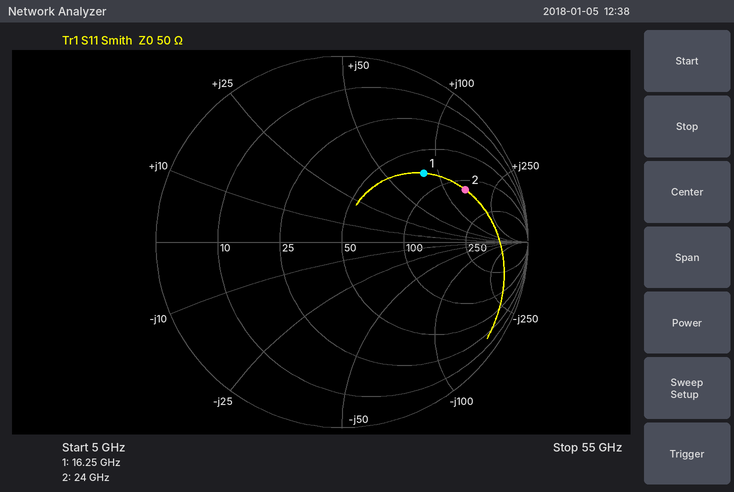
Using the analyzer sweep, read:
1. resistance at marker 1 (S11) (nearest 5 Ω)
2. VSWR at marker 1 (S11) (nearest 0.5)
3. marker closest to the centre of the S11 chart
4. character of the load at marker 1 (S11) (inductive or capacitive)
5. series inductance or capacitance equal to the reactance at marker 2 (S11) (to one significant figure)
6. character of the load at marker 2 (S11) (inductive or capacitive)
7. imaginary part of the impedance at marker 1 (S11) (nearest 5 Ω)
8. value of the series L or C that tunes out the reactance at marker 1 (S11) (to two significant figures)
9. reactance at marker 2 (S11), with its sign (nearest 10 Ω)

75 Ω
3.5
marker 1
inductive
1.0 nH
inductive
+80 Ω
120 fF
+150 Ω
